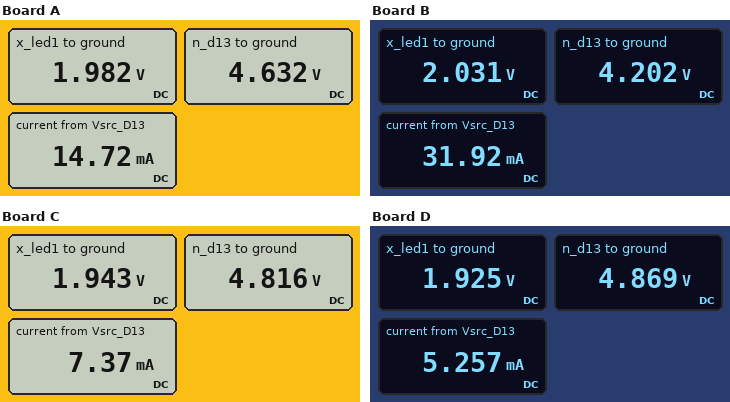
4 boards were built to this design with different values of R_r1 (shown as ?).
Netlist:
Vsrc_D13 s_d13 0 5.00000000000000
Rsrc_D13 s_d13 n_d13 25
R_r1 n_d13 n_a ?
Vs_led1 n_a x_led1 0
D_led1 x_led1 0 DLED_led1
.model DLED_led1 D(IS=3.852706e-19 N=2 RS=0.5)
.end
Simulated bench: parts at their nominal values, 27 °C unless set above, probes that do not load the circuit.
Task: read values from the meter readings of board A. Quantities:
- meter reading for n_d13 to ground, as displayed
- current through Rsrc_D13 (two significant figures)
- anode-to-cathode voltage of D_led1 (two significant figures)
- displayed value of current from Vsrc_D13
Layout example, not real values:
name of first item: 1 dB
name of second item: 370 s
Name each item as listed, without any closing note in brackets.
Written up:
meter reading for n_d13 to ground, as displayed: 4.632 V
current through Rsrc_D13: 15 mA
anode-to-cathode voltage of D_led1: 2.0 V
displayed value of current from Vsrc_D13: 14.72 mA
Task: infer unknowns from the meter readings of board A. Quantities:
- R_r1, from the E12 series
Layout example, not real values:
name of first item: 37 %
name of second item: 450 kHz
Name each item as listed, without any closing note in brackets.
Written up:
R_r1, from the E12 series: 180 Ω
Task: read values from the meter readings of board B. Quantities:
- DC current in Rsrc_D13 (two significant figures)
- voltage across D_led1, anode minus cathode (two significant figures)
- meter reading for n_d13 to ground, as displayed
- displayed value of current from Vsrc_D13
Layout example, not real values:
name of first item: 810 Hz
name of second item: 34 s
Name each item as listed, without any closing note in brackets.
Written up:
DC current in Rsrc_D13: 32 mA
voltage across D_led1, anode minus cathode: 2.0 V
meter reading for n_d13 to ground, as displayed: 4.202 V
displayed value of current from Vsrc_D13: 31.92 mA
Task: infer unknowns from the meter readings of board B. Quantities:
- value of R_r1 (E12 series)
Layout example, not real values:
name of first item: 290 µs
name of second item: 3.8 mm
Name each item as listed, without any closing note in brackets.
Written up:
value of R_r1: 68 Ω
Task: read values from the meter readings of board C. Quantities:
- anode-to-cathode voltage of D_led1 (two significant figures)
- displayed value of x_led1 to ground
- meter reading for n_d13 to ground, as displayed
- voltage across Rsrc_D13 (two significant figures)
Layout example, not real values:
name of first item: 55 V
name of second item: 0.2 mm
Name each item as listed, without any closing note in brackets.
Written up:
anode-to-cathode voltage of D_led1: 1.9 V
displayed value of x_led1 to ground: 1.943 V
meter reading for n_d13 to ground, as displayed: 4.816 V
voltage across Rsrc_D13: 180 mV
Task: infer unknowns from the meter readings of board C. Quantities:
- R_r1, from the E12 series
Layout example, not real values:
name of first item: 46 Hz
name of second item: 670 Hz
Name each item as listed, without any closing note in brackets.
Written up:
R_r1, from the E12 series: 390 Ω
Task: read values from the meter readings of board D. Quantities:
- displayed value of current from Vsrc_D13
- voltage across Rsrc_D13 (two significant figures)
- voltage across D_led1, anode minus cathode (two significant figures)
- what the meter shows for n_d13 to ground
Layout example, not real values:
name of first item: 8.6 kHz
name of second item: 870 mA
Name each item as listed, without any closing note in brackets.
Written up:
displayed value of current from Vsrc_D13: 5.257 mA
voltage across Rsrc_D13: 130 mV
voltage across D_led1, anode minus cathode: 1.9 V
what the meter shows for n_d13 to ground: 4.869 V
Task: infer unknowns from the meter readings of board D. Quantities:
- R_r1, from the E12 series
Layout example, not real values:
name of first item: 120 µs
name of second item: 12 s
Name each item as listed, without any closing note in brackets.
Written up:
R_r1, from the E12 series: 560 Ω
